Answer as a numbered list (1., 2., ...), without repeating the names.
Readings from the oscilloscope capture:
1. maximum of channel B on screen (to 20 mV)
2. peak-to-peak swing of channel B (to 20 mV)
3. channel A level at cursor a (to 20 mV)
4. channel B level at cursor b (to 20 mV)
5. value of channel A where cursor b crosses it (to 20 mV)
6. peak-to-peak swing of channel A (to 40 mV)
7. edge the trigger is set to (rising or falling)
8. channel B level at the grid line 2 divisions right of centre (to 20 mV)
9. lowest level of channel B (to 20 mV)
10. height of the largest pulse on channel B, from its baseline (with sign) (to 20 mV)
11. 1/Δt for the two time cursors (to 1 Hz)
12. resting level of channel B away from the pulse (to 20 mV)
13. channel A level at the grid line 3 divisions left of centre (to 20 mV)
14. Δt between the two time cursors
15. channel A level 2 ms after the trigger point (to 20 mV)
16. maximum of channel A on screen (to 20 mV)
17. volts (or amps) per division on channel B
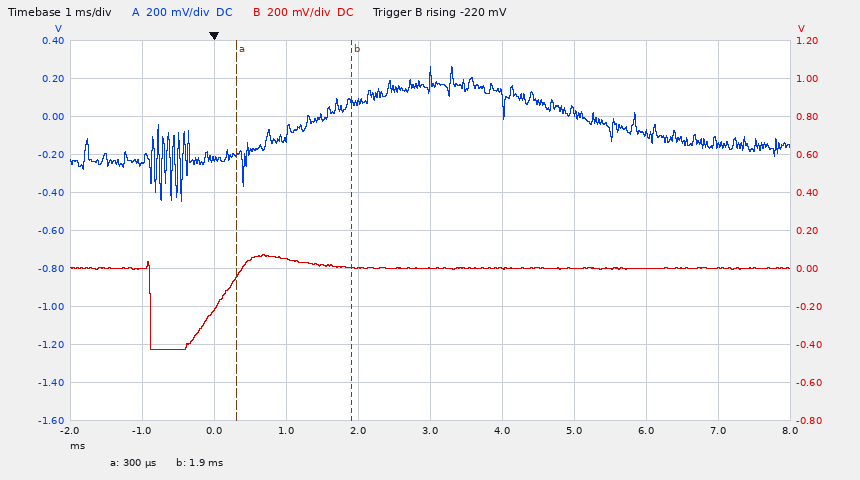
1. 80 mV
2. 500 mV
3. -200 mV
4. 0 mV
5. 80 mV
6. 720 mV
7. rising
8. 0 mV
9. -420 mV
10. -420 mV
11. 625 Hz
12. 0 mV
13. -220 mV
14. 1.6 ms
15. 80 mV
16. 260 mV
17. 200 mV
